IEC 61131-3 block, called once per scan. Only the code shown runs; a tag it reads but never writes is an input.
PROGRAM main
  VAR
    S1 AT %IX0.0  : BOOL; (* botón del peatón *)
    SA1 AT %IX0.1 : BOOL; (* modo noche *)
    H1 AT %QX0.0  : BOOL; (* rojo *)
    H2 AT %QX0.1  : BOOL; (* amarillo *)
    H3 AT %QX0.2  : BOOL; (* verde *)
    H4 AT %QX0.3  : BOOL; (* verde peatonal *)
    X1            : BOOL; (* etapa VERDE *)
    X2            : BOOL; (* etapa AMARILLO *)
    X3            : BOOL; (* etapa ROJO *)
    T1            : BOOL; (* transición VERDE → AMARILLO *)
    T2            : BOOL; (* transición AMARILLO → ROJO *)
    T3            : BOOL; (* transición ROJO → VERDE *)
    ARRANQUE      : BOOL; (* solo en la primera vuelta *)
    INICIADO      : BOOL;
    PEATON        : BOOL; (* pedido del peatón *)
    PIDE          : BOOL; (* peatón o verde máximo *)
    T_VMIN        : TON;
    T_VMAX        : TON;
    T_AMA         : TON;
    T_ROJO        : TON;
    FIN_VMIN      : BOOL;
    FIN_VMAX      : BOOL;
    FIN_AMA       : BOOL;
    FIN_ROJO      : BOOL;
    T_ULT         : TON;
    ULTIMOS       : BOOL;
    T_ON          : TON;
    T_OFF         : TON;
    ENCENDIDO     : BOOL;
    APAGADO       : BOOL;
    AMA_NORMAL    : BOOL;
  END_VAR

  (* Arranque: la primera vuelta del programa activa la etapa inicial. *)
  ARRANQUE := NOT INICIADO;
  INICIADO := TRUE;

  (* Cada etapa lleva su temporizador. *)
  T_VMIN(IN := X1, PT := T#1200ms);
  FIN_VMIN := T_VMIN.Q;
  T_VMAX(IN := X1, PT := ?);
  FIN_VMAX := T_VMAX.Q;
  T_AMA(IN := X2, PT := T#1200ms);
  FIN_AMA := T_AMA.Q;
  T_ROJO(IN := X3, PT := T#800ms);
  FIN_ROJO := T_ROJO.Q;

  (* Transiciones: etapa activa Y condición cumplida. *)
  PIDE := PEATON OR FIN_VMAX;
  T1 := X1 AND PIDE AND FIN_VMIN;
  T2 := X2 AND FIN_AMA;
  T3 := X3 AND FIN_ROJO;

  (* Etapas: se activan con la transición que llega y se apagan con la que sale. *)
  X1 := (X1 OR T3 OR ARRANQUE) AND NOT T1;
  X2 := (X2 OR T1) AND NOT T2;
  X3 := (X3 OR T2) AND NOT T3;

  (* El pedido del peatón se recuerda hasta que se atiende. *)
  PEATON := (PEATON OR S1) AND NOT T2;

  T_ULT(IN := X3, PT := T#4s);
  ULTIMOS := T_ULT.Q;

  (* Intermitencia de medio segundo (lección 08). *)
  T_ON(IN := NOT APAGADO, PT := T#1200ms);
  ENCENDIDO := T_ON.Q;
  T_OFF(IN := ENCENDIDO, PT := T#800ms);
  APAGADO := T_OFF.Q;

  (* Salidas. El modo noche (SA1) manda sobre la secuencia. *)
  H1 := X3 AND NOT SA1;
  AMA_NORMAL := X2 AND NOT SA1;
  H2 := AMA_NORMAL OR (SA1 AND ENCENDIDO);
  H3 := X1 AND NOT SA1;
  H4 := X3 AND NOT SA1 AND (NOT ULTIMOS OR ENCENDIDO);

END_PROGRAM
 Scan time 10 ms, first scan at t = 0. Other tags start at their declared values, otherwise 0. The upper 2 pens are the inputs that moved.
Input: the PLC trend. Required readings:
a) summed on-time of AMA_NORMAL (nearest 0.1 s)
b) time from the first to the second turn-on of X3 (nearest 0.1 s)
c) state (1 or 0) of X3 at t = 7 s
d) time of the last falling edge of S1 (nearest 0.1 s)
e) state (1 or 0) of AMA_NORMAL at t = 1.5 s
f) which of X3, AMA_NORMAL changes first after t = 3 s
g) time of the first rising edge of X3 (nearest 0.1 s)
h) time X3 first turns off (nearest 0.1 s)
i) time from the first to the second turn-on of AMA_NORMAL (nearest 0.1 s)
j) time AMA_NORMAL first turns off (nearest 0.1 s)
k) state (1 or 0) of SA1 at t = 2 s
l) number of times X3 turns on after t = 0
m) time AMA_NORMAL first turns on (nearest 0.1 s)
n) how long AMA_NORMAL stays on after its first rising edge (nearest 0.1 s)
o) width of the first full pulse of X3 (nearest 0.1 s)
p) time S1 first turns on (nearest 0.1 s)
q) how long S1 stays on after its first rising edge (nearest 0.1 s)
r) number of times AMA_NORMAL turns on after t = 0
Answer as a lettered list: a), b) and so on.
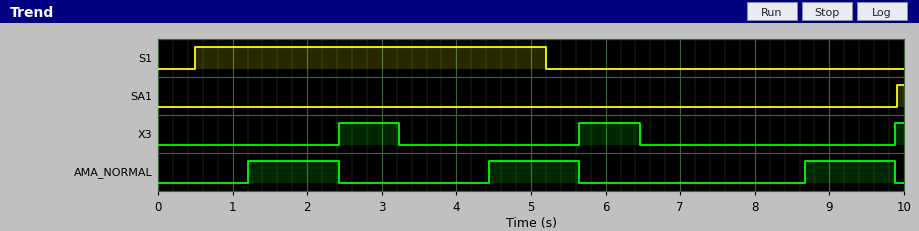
a) 3.6 s
b) 3.2 s
c) 0
d) 5.2 s
e) 1
f) X3
g) 2.4 s
h) 3.2 s
i) 3.2 s
j) 2.4 s
k) 0
l) 3
m) 1.2 s
n) 1.2 s
o) 0.8 s
p) 0.5 s
q) 4.7 s
r) 3
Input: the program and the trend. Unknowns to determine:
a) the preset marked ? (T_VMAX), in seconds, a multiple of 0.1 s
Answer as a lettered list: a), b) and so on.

a) 2.2 s
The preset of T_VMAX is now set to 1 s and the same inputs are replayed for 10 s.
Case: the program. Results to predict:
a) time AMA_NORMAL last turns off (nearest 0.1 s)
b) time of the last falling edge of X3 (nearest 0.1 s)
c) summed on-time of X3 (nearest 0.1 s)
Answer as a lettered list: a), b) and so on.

a) 8.9 s
b) 9.7 s
c) 2.4 s
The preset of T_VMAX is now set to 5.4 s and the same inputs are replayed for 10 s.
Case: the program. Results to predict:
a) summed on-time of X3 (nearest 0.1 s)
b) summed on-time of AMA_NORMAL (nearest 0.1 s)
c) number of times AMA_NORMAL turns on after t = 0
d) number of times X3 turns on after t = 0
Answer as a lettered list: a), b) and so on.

a) 1.6 s
b) 2.4 s
c) 2
d) 2
